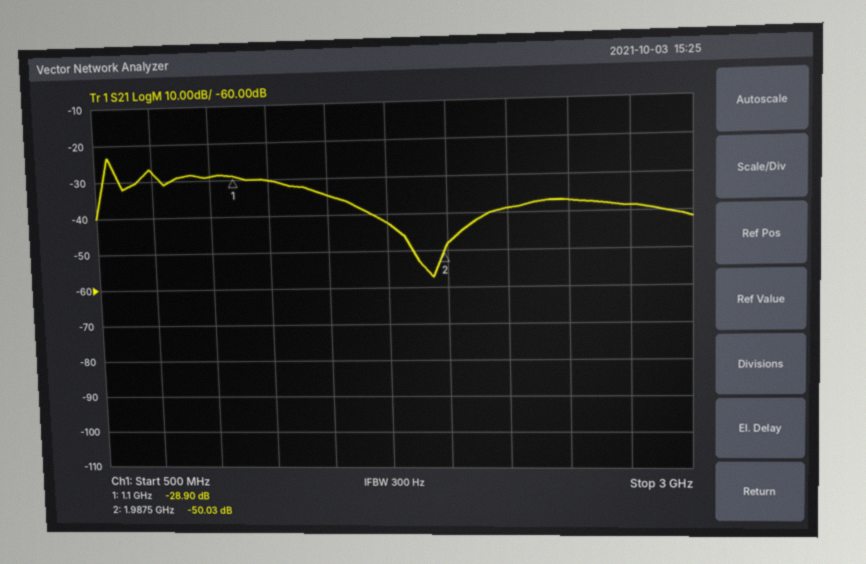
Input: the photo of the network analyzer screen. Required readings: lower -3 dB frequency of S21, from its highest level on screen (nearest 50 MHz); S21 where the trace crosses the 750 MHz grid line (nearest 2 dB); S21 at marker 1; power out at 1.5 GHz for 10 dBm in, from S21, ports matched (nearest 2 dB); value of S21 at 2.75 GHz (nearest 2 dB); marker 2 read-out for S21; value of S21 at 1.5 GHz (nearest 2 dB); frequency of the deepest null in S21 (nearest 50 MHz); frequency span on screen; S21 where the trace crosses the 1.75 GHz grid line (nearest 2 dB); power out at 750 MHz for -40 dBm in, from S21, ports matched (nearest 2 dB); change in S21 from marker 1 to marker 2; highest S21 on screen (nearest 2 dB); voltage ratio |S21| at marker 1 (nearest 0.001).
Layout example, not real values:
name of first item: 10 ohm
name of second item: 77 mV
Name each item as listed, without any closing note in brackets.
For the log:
lower -3 dB frequency of S21, from its highest level on screen: 550 MHz
S21 where the trace crosses the 750 MHz grid line: -28 dB
S21 at marker 1: -28.90 dB
power out at 1.5 GHz for 10 dBm in, from S21, ports matched: -24 dBm
value of S21 at 2.75 GHz: -38 dB
marker 2 read-out for S21: -50.03 dB
value of S21 at 1.5 GHz: -34 dB
frequency of the deepest null in S21: 1.95 GHz
frequency span on screen: 2.5 GHz
S21 where the trace crosses the 1.75 GHz grid line: -42 dB
power out at 750 MHz for -40 dBm in, from S21, ports matched: -68 dBm
change in S21 from marker 1 to marker 2: -21.13 dB
highest S21 on screen: -24 dB
voltage ratio |S21| at marker 1: 0.036
